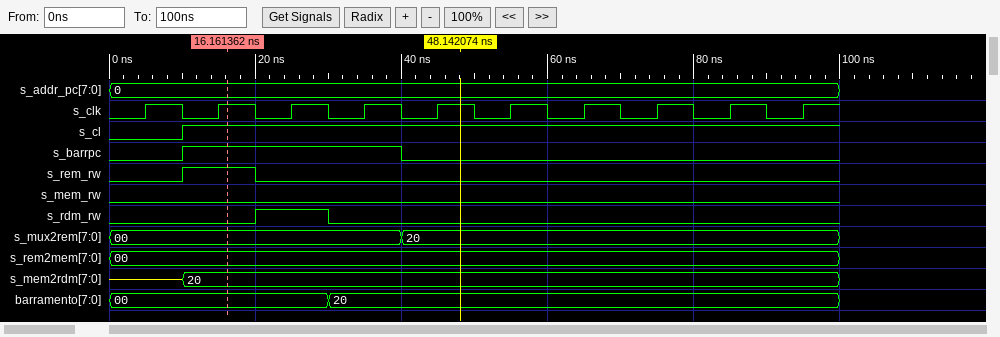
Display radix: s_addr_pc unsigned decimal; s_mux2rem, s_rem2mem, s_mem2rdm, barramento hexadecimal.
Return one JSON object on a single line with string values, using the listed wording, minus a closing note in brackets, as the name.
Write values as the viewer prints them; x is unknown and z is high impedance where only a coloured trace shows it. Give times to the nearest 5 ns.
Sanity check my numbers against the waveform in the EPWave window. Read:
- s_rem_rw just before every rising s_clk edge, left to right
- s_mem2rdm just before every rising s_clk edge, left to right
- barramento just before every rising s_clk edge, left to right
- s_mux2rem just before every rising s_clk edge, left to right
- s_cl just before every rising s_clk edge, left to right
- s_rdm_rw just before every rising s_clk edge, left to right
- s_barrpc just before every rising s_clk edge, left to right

{"s_rem_rw just before every rising s_clk edge, left to right": "0 1 0 0 0 0 0 0 0 0", "s_mem2rdm just before every rising s_clk edge, left to right": "z, 20, 20, 20, 20, 20, 20, 20, 20, 20", "barramento just before every rising s_clk edge, left to right": "00, 00, 00, 20, 20, 20, 20, 20, 20, 20", "s_mux2rem just before every rising s_clk edge, left to right": "00, 00, 00, 00, 20, 20, 20, 20, 20, 20", "s_cl just before every rising s_clk edge, left to right": "0 1 1 1 1 1 1 1 1 1", "s_rdm_rw just before every rising s_clk edge, left to right": "0 0 1 0 0 0 0 0 0 0", "s_barrpc just before every rising s_clk edge, left to right": "0 1 1 1 0 0 0 0 0 0"}
